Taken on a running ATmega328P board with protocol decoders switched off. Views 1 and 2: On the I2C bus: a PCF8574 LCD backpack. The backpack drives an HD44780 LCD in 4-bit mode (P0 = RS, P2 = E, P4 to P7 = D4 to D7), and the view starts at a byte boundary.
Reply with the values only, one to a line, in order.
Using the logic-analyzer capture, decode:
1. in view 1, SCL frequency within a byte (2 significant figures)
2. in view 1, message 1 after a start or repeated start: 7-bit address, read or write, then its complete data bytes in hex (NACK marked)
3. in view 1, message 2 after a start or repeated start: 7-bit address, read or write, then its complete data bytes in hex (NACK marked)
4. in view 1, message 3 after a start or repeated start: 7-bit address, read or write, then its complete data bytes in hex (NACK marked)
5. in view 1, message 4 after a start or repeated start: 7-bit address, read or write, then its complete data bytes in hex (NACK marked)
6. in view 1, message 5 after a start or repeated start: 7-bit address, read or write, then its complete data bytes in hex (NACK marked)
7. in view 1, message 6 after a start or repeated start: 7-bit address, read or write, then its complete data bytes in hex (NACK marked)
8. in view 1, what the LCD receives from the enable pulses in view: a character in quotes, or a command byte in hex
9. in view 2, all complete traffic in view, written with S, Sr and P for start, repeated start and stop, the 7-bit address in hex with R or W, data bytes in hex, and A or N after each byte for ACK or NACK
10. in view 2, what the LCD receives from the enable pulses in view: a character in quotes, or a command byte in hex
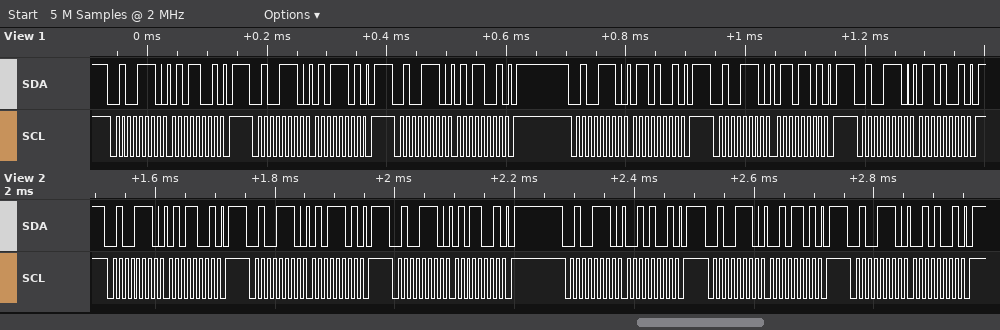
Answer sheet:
100 kHz
0x27 write: 59
0x27 write: 5D
0x27 write: 59
0x27 write: 69
0x27 write: 6D
0x27 write: 69
'V'
S 27W A 59 A P S 27W A 5D A P S 27W A 59 A P S 27W A 29 A P S 27W A 2D A P S 27W A 29 A P
'R'
